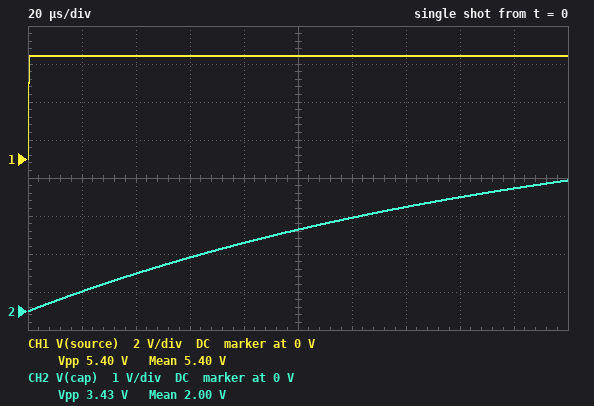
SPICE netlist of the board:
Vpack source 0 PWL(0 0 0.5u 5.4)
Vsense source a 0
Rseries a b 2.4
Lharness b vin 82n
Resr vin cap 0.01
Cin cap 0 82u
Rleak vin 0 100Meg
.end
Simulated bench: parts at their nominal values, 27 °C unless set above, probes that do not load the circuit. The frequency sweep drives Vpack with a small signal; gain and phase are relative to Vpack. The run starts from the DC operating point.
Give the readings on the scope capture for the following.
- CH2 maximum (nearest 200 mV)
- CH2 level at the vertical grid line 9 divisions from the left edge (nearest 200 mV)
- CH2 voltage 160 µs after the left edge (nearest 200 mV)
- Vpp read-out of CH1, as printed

3.4 V
3.2 V
3.0 V
5.40 V
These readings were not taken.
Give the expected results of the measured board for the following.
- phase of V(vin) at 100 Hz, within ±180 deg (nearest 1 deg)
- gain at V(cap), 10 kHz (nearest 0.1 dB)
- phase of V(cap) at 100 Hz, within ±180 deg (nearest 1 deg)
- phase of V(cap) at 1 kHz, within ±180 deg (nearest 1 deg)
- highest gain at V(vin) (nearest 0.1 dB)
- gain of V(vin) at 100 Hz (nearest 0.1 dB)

-7 deg
-21.9 dB
-7 deg
-51 deg
0 dB
-0.1 dB
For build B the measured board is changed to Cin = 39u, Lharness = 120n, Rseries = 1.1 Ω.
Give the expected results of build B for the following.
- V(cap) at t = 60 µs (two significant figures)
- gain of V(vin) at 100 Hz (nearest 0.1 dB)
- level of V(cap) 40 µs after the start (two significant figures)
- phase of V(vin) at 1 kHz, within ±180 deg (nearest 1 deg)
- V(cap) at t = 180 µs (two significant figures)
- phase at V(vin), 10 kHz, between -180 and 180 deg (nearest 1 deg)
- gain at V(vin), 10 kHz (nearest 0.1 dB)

4.0 V
0 dB
3.2 V
-15 deg
5.3 V
-69 deg
-9.2 dB
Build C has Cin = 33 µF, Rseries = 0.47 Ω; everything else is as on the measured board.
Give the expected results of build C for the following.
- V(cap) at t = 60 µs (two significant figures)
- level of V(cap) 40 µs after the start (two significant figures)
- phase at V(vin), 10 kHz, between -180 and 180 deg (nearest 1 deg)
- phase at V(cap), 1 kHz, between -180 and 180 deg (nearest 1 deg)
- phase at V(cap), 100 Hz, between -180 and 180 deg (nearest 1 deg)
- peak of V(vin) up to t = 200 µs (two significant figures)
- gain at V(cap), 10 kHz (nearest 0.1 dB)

5.3 V
5.0 V
-44 deg
-6 deg
-1 deg
5.4 V
-2.9 dB
